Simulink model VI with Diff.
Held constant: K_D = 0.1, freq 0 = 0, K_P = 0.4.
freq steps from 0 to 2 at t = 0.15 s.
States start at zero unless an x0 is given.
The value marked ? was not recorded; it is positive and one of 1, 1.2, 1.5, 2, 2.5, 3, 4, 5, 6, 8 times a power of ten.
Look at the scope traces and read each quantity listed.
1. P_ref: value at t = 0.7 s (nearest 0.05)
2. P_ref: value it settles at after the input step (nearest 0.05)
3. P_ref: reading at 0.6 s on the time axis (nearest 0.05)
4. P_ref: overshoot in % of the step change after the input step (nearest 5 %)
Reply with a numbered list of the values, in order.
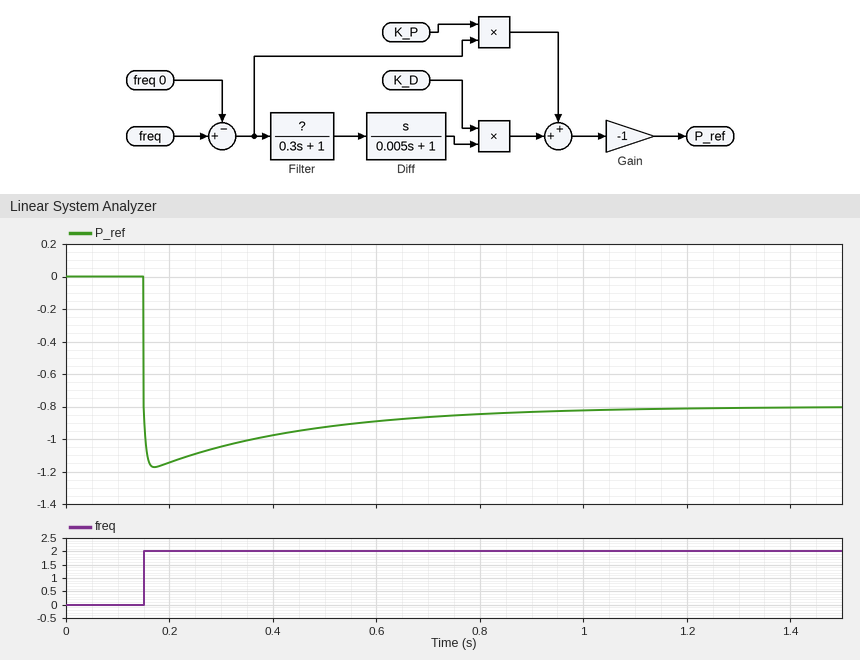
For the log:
1. -0.85
2. -0.80
3. -0.90
4. 45 %
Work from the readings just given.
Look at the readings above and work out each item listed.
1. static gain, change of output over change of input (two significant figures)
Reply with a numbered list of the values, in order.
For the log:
1. -0.40
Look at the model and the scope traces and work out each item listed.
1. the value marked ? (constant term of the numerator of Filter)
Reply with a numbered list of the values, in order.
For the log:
1. 0.6
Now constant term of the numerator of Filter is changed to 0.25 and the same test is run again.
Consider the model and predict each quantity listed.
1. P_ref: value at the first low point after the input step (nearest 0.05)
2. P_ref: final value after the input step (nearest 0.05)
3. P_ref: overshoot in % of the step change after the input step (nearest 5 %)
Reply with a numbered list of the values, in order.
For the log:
1. -0.95
2. -0.80
3. 20 %
